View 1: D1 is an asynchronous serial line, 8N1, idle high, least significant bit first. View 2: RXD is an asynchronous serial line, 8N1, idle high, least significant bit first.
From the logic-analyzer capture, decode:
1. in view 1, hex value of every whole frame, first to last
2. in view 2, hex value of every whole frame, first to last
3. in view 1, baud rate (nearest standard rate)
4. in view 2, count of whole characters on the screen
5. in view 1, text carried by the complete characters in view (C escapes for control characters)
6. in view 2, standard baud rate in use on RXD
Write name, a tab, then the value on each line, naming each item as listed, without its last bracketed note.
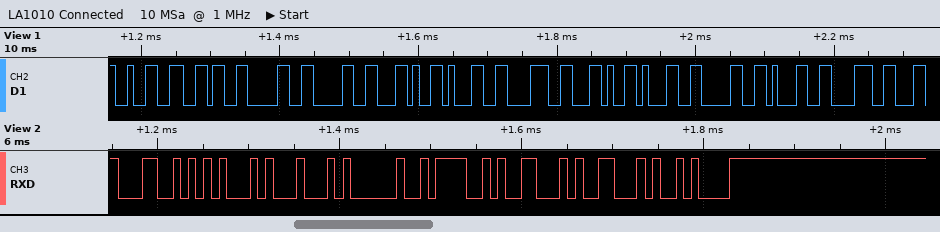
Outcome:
in view 1, hex value of every whole frame, first to last	0x32 0x36 0x30 0x30 0x2C 0x31 0x38 0x2C 0x31 0x30 0x31 0x38
in view 2, hex value of every whole frame, first to last	0x4C 0x45 0x44 0x20 0x4F 0x46 0x46 0x0A
in view 1, baud rate	115200 baud
in view 2, count of whole characters on the screen	8
in view 1, text carried by the complete characters in view	"2600,18,1018"
in view 2, standard baud rate in use on RXD	115200 baud
